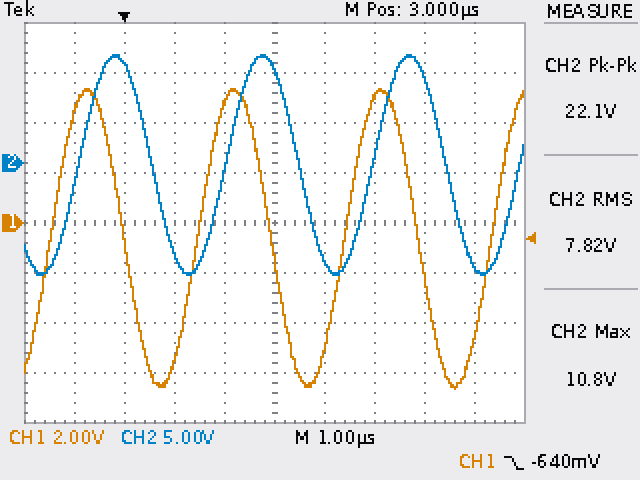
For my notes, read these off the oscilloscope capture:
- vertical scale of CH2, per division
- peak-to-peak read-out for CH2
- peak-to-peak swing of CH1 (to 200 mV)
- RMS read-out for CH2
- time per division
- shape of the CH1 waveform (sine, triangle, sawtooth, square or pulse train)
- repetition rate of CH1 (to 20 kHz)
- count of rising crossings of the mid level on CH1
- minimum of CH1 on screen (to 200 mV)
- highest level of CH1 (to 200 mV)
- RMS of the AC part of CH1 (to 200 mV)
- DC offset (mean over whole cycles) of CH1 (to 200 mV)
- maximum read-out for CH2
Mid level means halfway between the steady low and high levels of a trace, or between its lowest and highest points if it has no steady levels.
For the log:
5 V
22.1 V
12.0 V
7.82 V
1 µs
sine
340 kHz
4
-6.6 V
5.4 V
4.2 V
-600 mV
10.8 V
